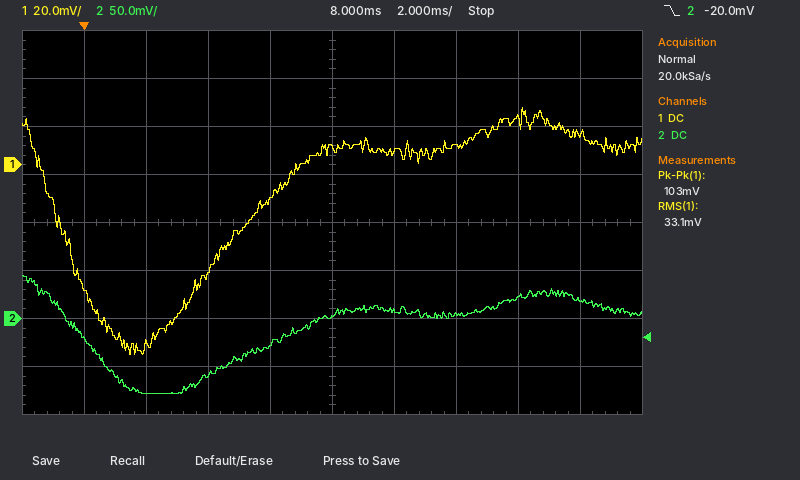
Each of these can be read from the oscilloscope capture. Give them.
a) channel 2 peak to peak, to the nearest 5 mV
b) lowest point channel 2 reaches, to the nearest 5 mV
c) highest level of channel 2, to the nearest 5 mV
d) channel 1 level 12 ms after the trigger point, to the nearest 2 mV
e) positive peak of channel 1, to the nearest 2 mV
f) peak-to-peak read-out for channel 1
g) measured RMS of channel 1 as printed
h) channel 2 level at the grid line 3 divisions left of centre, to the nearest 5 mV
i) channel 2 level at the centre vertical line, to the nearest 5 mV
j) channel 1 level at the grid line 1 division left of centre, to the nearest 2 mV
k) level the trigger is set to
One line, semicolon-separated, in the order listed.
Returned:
125 mV; -80 mV; 45 mV; 8 mV; 24 mV; 103 mV; 33.1 mV; -80 mV; 0 mV; -14 mV; -20.0 mV
